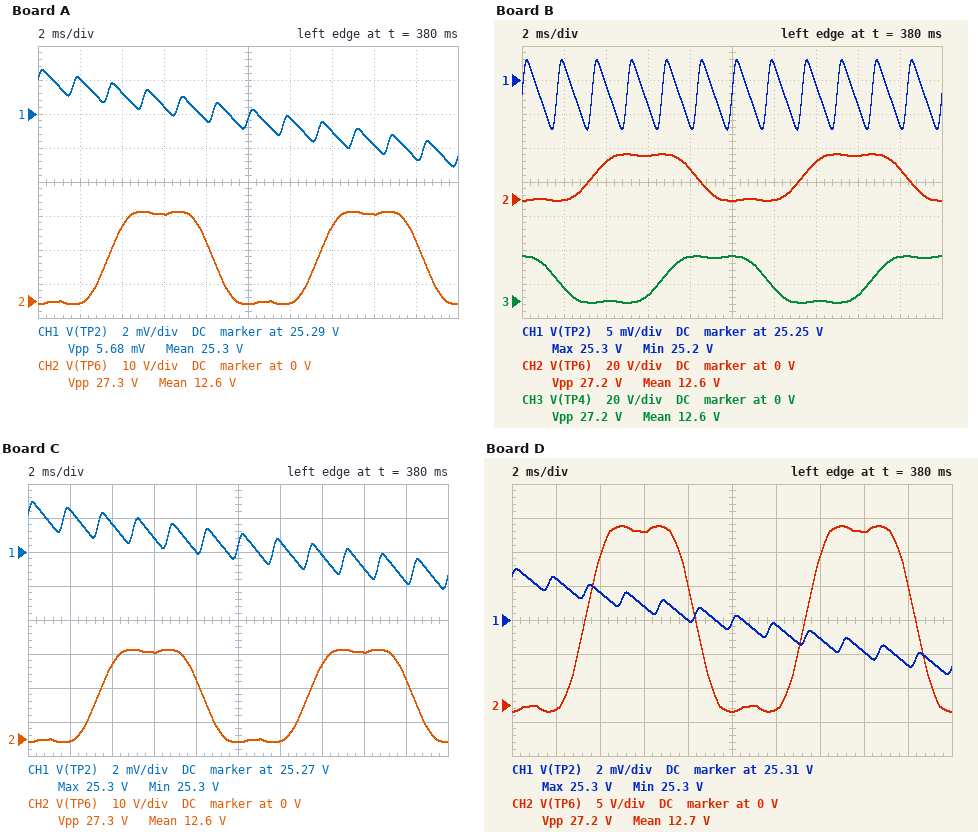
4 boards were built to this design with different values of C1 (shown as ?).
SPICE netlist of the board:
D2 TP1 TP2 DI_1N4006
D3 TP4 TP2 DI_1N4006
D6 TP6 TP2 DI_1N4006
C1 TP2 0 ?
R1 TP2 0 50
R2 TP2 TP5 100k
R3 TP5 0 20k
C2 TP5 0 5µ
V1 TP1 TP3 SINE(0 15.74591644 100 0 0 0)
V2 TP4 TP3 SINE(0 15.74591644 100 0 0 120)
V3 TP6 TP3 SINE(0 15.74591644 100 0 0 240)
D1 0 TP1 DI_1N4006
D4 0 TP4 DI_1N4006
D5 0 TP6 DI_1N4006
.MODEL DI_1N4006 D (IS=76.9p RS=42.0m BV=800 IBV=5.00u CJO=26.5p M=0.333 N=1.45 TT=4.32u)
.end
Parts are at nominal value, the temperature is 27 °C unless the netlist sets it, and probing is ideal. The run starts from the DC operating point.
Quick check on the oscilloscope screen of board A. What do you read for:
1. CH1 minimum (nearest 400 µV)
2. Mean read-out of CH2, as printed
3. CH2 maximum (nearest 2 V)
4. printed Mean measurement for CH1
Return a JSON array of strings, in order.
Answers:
["25.2848 V", "12.6 V", "26 V", "25.3 V"]
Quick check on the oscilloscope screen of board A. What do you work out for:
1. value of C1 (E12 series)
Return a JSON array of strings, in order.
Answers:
["390 mF"]
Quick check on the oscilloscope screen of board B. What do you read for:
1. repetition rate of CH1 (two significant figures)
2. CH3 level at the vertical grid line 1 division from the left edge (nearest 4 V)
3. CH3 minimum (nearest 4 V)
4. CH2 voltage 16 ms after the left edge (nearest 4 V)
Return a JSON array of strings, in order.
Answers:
["600 Hz", "8 V", "0 V", "24 V"]
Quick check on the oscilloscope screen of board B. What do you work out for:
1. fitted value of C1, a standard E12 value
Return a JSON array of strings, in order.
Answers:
["56 mF"]
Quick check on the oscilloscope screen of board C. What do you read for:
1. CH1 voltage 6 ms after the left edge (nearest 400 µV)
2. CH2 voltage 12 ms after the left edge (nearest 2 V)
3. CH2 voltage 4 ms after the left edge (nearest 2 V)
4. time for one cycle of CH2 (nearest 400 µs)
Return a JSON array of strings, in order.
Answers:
["25.2748 V", "0 V", "22 V", "10.0 ms"]
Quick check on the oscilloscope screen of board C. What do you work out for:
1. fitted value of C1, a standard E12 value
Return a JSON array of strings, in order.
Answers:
["330 mF"]
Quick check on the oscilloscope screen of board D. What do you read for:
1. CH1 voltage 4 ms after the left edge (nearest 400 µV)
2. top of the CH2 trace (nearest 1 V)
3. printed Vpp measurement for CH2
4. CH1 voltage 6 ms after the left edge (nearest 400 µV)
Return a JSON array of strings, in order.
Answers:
["25.3076 V", "26 V", "27.2 V", "25.3068 V"]
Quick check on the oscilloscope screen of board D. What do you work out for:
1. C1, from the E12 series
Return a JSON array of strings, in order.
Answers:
["470 mF"]
